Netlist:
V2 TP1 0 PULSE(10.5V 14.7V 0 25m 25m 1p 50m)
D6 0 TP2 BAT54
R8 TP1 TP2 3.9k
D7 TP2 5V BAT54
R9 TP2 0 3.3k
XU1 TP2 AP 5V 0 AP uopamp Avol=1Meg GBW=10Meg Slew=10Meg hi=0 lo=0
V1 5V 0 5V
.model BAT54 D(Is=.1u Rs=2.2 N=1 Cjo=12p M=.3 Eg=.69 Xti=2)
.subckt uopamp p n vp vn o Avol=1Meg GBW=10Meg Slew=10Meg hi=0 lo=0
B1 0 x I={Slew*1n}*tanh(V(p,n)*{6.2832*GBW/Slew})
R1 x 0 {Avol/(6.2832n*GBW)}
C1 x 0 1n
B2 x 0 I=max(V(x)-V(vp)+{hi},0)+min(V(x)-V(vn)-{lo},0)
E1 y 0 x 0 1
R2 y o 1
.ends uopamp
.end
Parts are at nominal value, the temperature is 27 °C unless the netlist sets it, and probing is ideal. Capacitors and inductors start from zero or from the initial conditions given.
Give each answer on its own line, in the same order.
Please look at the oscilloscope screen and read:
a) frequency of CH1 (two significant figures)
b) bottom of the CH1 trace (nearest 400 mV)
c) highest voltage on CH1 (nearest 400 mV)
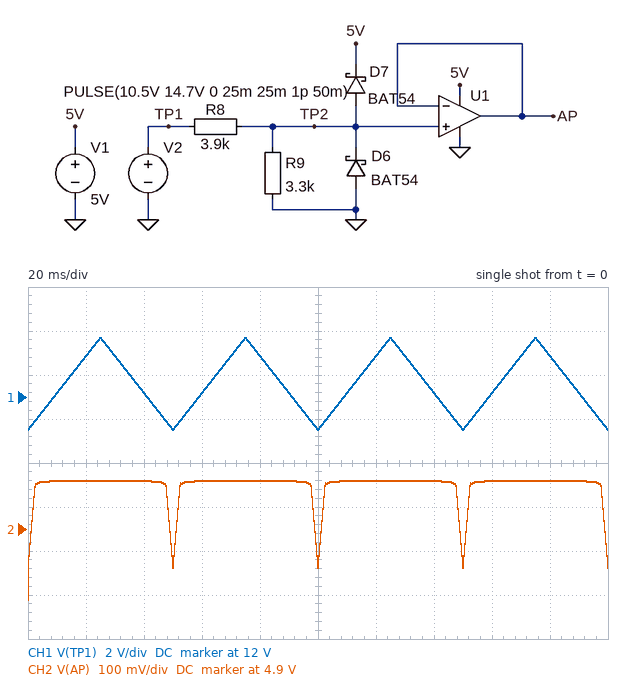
20 Hz
10.4 V
14.8 V
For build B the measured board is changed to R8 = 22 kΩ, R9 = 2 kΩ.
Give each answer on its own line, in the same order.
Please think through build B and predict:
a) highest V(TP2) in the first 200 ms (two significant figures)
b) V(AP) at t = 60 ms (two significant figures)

1.2 V
1.0 V
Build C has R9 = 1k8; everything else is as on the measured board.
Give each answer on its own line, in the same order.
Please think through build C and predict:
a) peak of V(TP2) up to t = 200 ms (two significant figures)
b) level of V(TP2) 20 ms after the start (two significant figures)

4.6 V
4.4 V
